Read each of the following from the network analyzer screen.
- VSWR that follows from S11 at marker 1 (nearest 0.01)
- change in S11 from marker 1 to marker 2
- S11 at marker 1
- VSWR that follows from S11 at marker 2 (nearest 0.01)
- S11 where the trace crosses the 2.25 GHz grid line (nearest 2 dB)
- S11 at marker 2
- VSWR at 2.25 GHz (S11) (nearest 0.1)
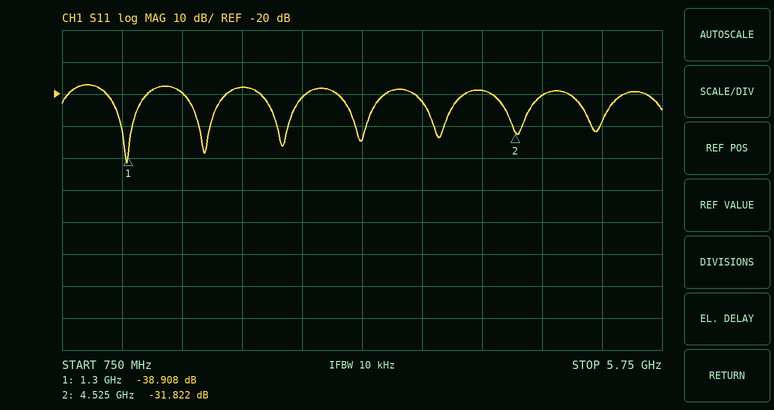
1.02
7.086 dB
-38.908 dB
1.05
-18 dB
-31.822 dB
1.3
